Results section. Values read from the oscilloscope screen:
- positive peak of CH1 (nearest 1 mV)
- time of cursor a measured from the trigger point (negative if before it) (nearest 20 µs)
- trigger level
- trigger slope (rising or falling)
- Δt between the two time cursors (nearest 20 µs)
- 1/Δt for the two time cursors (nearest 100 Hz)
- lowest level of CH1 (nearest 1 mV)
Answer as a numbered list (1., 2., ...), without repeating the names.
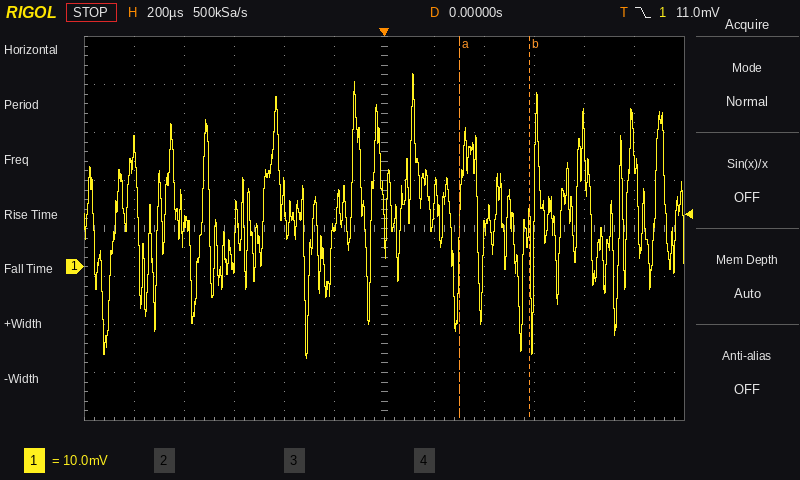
1. 40 mV
2. +300 µs
3. 11.0 mV
4. falling
5. 280 µs
6. 3.6 kHz
7. -19 mV
